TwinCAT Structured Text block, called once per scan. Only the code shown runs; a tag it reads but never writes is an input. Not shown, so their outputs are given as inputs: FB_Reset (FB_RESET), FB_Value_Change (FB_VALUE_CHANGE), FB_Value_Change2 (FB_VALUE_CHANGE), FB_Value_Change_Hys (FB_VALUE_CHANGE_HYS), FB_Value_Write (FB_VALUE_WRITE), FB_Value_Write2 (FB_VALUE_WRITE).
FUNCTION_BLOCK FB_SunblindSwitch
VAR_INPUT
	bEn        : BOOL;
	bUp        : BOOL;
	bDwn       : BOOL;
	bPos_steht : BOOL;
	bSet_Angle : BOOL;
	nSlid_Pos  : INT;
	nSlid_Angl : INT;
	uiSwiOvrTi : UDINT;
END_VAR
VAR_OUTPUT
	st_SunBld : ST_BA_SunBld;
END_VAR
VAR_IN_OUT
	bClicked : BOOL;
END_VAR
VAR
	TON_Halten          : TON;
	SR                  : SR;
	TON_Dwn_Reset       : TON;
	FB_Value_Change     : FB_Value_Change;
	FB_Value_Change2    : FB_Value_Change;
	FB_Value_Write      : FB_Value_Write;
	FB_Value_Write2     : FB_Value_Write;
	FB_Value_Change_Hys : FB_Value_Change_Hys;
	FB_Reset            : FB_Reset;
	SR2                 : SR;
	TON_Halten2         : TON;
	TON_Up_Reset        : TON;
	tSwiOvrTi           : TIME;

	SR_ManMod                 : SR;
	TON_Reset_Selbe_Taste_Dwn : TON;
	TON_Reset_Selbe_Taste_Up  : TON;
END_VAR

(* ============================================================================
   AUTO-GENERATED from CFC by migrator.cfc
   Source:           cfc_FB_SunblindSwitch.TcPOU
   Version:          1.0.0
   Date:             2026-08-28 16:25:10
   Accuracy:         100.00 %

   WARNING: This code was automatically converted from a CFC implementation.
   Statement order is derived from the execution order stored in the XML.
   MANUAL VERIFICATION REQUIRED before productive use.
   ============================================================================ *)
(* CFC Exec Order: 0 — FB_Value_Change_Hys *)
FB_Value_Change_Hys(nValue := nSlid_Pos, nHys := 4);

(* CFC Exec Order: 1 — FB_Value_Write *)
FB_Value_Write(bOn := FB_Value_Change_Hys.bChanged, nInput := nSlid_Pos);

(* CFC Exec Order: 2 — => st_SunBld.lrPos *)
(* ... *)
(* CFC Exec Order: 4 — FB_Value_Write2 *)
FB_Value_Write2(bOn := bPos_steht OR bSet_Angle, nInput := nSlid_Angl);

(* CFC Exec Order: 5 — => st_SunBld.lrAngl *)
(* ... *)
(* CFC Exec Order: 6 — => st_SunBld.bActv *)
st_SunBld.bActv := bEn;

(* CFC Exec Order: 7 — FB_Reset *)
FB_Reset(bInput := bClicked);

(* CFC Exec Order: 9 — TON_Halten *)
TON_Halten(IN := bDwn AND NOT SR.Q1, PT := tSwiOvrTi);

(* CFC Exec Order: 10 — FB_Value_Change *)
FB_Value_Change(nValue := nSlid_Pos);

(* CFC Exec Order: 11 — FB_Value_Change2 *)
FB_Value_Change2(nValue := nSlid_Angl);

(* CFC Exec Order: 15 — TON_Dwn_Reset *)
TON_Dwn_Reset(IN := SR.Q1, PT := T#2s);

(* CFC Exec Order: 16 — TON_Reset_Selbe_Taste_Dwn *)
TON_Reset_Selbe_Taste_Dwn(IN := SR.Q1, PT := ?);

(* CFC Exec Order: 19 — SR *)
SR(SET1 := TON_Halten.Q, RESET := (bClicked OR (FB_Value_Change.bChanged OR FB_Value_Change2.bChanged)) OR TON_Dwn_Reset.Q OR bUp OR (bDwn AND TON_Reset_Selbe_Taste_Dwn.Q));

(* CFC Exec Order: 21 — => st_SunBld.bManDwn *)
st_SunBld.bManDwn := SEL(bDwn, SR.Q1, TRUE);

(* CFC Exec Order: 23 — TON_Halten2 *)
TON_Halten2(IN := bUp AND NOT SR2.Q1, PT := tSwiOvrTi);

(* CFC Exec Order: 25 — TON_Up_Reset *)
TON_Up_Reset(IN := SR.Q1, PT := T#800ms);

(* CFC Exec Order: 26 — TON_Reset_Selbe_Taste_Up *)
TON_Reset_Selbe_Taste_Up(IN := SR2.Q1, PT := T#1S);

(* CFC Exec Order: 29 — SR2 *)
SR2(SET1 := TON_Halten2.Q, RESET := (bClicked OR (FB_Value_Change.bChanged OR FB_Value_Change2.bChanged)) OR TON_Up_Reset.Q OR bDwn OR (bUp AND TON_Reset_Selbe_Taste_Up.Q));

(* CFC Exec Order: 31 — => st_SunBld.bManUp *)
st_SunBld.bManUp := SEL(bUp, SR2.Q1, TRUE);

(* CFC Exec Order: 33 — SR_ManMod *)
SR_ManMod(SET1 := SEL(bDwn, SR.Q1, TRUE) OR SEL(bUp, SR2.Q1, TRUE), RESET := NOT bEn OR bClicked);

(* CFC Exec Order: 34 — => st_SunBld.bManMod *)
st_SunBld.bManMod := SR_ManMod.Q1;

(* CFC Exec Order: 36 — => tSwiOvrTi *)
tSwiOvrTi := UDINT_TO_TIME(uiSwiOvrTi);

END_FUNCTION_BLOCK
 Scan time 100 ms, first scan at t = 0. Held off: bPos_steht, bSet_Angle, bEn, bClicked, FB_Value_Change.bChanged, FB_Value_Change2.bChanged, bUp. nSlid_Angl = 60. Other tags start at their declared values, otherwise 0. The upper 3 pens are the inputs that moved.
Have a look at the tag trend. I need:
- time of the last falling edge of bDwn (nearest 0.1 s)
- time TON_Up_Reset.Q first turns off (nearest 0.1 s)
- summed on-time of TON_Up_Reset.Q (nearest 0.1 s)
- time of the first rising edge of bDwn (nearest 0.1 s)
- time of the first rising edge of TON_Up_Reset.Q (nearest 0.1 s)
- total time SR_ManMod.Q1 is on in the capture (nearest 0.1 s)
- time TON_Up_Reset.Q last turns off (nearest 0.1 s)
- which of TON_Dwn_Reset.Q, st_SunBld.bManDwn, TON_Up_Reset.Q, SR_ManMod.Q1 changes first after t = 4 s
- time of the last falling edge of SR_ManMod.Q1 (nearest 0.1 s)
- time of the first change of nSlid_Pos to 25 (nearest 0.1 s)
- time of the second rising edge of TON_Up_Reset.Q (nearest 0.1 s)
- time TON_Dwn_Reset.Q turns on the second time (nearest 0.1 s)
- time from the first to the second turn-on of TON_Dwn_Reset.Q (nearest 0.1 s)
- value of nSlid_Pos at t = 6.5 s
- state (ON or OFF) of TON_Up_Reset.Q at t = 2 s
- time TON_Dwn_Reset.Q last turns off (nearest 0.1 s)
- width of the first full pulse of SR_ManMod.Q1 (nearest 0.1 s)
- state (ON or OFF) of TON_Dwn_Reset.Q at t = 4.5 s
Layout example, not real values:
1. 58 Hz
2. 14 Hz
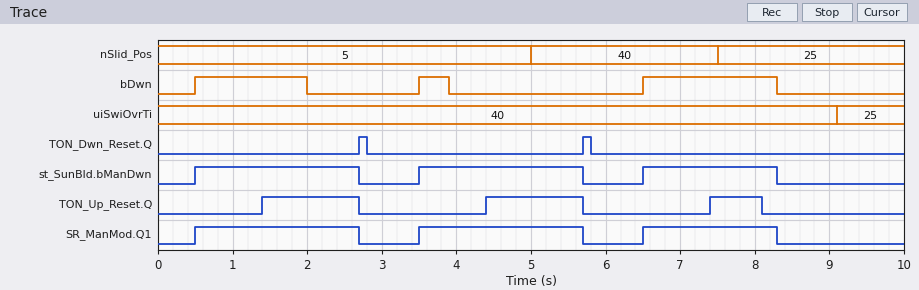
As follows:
1. 8.3 s
2. 2.7 s
3. 3.3 s
4. 0.5 s
5. 1.4 s
6. 6.2 s
7. 8.1 s
8. TON_Up_Reset.Q
9. 8.3 s
10. 7.5 s
11. 4.4 s
12. 5.7 s
13. 3.0 s
14. 40
15. ON
16. 5.8 s
17. 2.2 s
18. OFF
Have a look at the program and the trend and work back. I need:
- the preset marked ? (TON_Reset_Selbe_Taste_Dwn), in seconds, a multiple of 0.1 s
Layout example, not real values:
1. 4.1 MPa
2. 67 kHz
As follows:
1. 1.4 s
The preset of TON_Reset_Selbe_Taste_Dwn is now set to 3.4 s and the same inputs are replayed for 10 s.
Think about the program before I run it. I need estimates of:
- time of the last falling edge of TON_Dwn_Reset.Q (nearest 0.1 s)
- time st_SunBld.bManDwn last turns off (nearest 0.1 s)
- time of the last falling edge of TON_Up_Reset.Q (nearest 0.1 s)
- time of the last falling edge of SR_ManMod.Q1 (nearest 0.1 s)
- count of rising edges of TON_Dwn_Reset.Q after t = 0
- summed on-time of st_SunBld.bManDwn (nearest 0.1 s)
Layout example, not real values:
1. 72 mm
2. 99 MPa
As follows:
1. 8.8 s
2. 8.7 s
3. 8.7 s
4. 8.7 s
5. 3
6. 6.6 s
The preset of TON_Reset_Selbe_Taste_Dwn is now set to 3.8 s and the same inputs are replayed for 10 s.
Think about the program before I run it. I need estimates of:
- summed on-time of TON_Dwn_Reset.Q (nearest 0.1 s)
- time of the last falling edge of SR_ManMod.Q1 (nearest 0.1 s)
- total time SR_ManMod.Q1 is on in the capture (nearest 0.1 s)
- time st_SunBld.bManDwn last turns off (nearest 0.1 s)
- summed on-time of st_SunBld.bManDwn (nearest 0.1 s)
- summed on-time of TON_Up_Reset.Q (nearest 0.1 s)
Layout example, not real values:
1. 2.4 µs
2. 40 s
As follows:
1. 0.3 s
2. 8.7 s
3. 6.6 s
4. 8.7 s
5. 6.6 s
6. 3.9 s
